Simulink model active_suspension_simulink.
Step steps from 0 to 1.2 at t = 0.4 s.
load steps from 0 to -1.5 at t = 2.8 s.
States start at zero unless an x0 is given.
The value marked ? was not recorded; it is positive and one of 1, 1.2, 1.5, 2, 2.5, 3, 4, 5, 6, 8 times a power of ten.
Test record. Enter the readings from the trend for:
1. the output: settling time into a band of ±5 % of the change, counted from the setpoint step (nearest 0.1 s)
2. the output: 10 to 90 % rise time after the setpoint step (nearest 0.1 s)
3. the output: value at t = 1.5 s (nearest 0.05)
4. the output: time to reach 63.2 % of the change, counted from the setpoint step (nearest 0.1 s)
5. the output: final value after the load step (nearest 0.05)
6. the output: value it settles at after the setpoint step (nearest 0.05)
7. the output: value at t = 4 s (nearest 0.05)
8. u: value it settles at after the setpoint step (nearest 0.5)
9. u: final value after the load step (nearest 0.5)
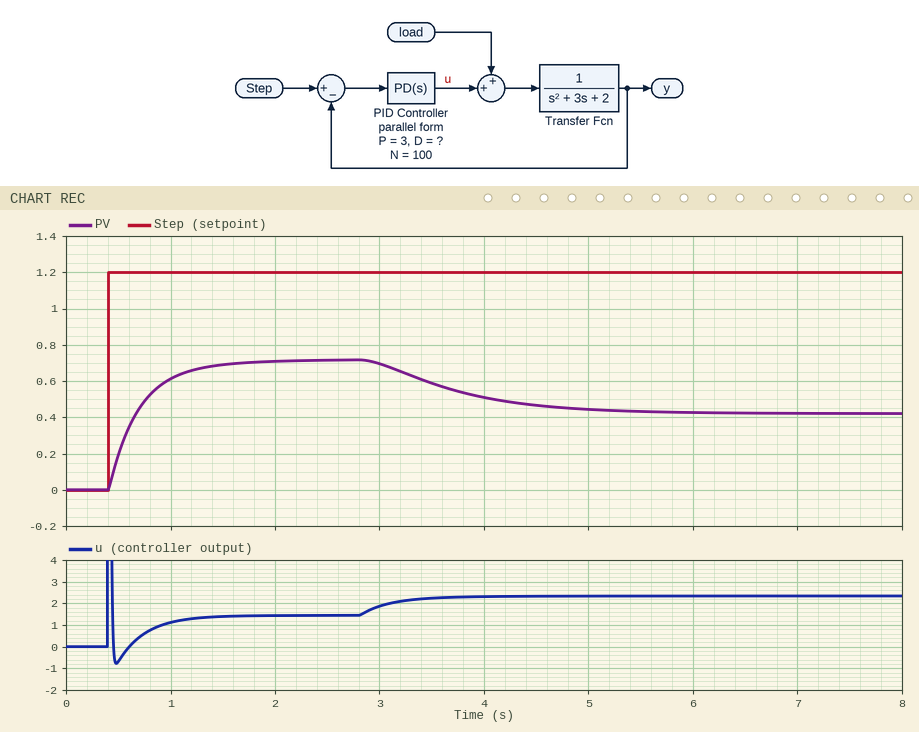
1.0 s
0.7 s
0.70
0.3 s
0.40
0.70
0.50
1.5
2.5
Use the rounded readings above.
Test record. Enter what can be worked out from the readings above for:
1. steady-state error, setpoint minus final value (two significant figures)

0.50
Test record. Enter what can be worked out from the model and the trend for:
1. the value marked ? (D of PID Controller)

2
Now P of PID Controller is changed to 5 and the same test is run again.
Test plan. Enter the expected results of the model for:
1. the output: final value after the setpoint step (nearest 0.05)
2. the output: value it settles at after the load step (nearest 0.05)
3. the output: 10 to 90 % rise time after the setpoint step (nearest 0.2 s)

0.85
0.65
0.6 s
